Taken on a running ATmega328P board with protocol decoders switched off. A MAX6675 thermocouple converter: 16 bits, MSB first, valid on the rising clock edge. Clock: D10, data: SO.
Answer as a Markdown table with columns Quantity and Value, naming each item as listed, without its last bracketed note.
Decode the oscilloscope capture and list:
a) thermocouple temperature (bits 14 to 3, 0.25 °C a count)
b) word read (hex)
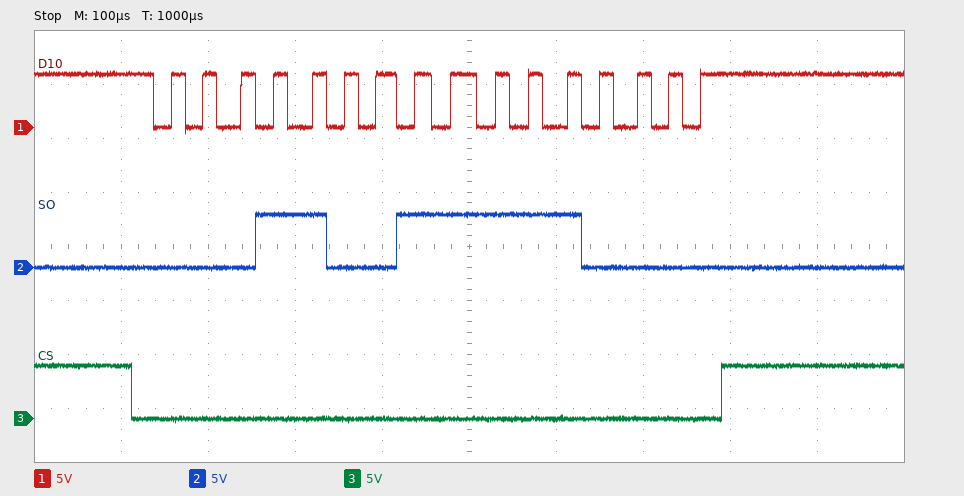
| Quantity | Value |
|---|---|
| thermocouple temperature | 207.50 °C |
| word read | 0x19F0 |
